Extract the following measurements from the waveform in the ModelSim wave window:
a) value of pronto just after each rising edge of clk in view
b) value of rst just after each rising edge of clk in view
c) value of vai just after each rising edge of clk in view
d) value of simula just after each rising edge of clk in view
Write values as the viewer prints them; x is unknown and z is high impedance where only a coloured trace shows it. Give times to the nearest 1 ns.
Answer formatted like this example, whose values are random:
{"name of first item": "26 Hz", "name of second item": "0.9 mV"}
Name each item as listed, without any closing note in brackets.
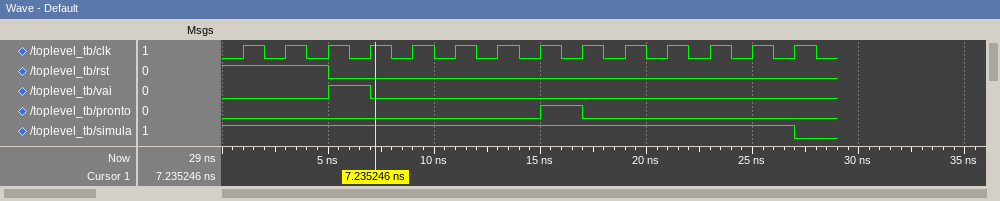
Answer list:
{"value of pronto just after each rising edge of clk in view": "0 0 0 0 0 0 0 1 0 0 0 0 0 0", "value of rst just after each rising edge of clk in view": "1 1 0 0 0 0 0 0 0 0 0 0 0 0", "value of vai just after each rising edge of clk in view": "0 0 1 0 0 0 0 0 0 0 0 0 0 0", "value of simula just after each rising edge of clk in view": "1 1 1 1 1 1 1 1 1 1 1 1 1 0"}
